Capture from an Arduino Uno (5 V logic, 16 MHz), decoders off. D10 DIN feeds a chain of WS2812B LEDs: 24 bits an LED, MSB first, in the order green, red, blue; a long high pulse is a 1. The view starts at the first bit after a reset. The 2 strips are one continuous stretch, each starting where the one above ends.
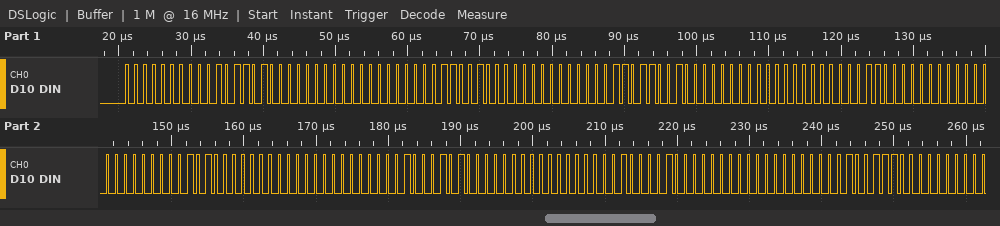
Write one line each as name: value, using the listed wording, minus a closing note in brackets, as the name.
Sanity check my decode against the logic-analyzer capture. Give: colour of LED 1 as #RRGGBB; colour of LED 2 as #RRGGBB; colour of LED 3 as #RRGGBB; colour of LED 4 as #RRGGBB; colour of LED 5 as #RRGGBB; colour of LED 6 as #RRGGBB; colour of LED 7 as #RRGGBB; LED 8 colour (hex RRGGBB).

colour of LED 1 as #RRGGBB: #2D0000
colour of LED 2 as #RRGGBB: #190000
colour of LED 3 as #RRGGBB: #640300
colour of LED 4 as #RRGGBB: #300000
colour of LED 5 as #RRGGBB: #500000
colour of LED 6 as #RRGGBB: #450000
colour of LED 7 as #RRGGBB: #420000
LED 8 colour: #270000
